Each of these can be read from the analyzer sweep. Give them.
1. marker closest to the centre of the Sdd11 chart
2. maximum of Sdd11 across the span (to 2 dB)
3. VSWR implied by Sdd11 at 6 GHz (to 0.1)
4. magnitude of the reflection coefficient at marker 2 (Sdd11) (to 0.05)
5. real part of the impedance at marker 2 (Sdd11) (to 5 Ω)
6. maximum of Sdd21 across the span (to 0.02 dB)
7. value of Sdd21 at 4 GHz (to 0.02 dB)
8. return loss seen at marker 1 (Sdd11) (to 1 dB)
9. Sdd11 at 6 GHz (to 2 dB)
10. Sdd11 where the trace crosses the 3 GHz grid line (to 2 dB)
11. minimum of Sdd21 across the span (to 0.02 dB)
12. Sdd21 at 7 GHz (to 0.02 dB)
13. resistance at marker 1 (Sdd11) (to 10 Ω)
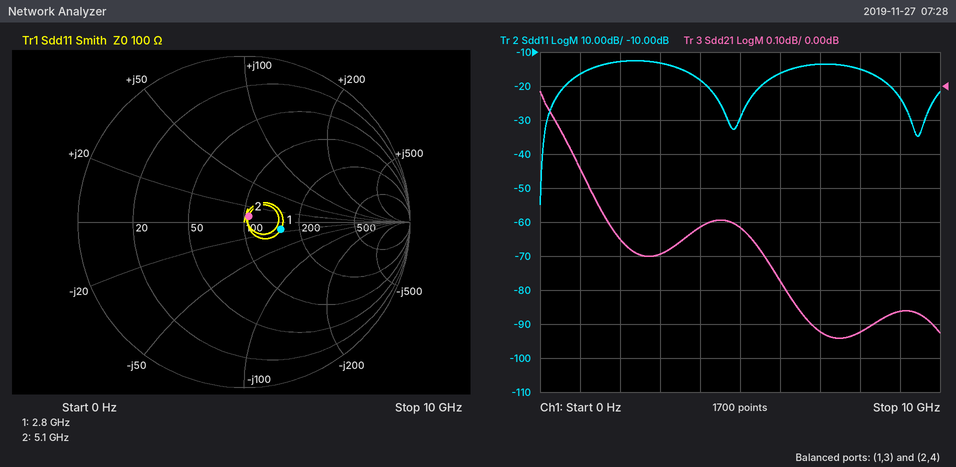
marker 2
-12 dB
1.4
0.05
105 Ω
-0.02 dB
-0.42 dB
13 dB
-16 dB
-14 dB
-0.74 dB
-0.72 dB
160 Ω
